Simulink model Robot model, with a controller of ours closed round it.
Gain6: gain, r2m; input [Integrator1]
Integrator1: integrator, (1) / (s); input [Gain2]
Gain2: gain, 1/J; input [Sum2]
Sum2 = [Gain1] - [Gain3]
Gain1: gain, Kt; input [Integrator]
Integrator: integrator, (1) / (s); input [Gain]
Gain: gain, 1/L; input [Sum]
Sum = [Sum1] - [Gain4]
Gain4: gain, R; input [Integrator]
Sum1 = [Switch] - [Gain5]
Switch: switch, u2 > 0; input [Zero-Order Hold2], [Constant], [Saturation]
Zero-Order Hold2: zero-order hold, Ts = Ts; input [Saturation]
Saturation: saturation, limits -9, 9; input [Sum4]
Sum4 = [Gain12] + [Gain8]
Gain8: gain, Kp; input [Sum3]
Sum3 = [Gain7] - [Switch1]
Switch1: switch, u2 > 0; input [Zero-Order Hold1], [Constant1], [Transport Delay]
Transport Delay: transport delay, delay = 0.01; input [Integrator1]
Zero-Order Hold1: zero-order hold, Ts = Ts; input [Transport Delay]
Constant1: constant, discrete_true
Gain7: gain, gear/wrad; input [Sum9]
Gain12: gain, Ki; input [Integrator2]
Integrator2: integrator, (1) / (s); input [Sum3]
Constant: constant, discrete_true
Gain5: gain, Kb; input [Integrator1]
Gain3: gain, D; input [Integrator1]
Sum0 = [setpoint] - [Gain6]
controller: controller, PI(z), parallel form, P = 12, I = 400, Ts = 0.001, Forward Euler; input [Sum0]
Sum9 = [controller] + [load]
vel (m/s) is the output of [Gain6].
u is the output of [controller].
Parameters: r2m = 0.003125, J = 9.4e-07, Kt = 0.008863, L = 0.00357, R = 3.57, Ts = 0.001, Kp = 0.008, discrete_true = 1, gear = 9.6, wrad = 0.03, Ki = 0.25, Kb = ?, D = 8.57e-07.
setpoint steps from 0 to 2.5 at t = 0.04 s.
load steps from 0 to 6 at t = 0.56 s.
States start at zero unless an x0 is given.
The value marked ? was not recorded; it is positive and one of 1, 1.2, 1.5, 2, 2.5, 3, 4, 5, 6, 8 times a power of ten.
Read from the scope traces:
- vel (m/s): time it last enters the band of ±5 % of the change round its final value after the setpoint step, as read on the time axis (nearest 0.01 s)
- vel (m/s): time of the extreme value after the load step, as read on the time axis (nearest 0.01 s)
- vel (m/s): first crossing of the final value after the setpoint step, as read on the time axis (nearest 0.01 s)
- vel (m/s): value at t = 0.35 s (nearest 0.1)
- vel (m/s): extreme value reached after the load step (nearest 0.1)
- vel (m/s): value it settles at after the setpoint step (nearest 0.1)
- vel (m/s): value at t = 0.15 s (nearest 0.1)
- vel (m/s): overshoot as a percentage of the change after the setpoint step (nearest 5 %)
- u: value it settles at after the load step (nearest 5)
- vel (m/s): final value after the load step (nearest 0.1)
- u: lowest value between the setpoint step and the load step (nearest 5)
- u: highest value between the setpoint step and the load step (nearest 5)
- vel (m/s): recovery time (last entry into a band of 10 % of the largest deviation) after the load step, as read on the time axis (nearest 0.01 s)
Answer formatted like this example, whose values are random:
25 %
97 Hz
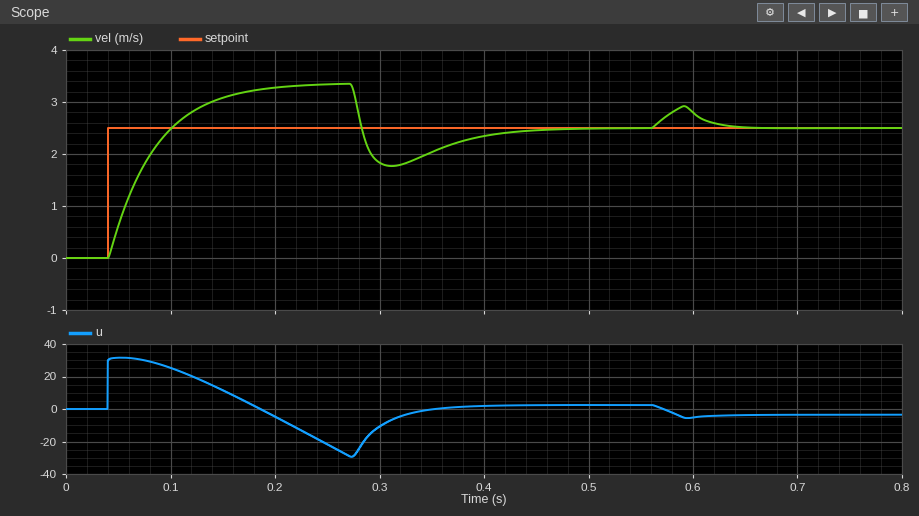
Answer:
0.41 s
0.59 s
0.10 s
2.0
2.9
2.5
3.1
35 %
-5
2.5
-30
30
0.63 s
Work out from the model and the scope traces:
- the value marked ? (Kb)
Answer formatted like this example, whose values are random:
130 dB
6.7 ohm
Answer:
0.008
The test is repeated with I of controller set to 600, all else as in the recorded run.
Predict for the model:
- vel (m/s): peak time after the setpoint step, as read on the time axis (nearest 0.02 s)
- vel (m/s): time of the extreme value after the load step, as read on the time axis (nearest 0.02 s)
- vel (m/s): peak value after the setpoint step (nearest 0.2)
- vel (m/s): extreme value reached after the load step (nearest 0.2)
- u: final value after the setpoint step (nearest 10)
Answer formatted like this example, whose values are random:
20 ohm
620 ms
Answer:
0.28 s
0.58 s
3.4
2.8
0
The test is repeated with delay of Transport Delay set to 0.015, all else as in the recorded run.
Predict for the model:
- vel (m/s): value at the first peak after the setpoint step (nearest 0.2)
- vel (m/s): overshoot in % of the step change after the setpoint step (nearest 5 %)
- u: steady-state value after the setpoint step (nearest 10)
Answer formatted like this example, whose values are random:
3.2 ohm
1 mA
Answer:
3.4
35 %
0
